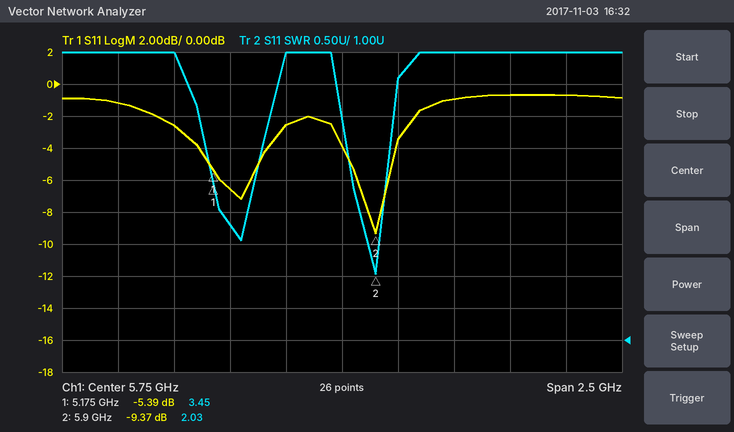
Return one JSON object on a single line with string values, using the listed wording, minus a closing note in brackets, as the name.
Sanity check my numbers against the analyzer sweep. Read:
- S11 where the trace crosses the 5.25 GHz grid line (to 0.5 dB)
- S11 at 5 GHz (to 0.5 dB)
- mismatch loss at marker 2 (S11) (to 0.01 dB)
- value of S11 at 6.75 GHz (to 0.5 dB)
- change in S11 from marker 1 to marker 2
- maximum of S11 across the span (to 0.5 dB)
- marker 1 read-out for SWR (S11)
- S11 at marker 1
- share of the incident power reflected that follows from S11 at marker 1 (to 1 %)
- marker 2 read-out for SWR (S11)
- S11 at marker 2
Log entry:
{"S11 where the trace crosses the 5.25 GHz grid line": "-6.5 dB", "S11 at 5 GHz": "-2.5 dB", "mismatch loss at marker 2 (S11)": "0.53 dB", "value of S11 at 6.75 GHz": "-0.5 dB", "change in S11 from marker 1 to marker 2": "-3.98 dB", "maximum of S11 across the span": "-0.5 dB", "marker 1 read-out for SWR": "3.45", "S11 at marker 1": "-5.39 dB", "share of the incident power reflected that follows from S11 at marker 1": "29 %", "marker 2 read-out for SWR": "2.03", "S11 at marker 2": "-9.37 dB"}
